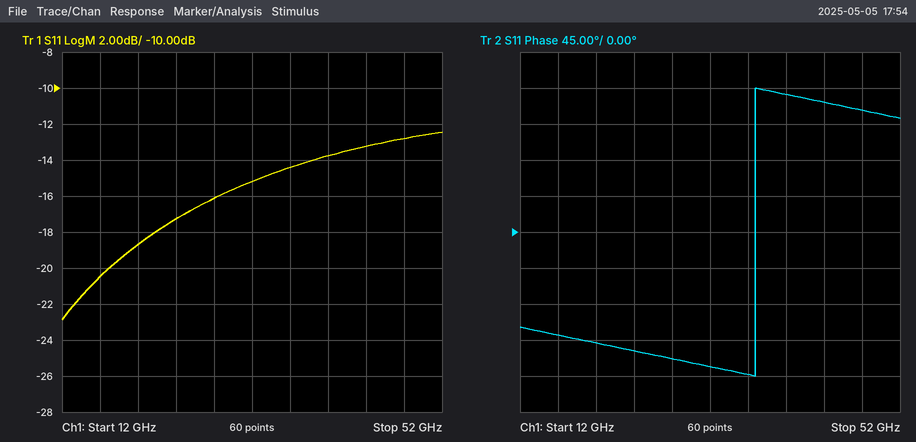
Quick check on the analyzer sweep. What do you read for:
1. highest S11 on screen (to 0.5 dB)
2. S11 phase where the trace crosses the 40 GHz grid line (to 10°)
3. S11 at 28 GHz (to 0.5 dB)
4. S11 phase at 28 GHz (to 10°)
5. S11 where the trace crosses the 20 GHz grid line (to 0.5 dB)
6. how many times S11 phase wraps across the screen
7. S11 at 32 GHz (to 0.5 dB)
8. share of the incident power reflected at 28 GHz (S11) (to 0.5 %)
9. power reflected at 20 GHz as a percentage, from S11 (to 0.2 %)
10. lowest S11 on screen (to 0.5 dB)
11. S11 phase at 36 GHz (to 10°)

-12.5 dB
170°
-16.0 dB
-160°
-18.5 dB
1
-15.0 dB
2.5 %
1.4 %
-23.0 dB
-180°
